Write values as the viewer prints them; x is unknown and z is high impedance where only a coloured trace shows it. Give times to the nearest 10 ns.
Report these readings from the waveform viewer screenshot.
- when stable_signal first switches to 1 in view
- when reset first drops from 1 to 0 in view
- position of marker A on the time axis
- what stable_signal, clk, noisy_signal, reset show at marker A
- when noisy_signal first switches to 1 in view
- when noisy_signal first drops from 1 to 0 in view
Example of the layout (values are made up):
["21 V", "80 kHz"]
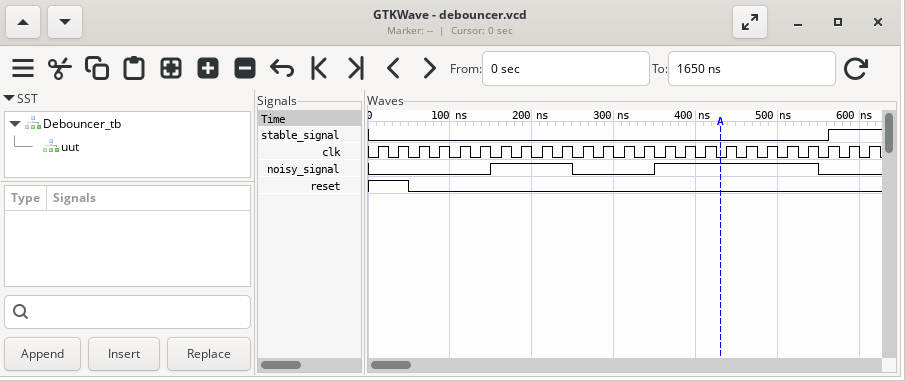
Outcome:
["560 ns", "50 ns", "430 ns", "stable_signal=0, clk=0, noisy_signal=1, reset=0", "150 ns", "250 ns"]
